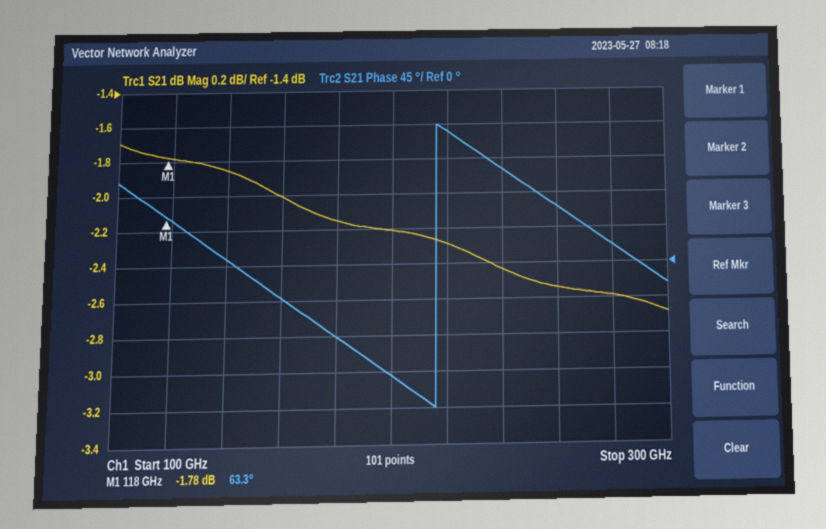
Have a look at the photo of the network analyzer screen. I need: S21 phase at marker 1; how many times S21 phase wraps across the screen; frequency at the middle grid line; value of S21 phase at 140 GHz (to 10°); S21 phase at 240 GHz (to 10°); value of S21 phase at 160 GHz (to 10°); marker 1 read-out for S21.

63.3°
1
200 GHz
10°
120°
-40°
-1.78 dB
